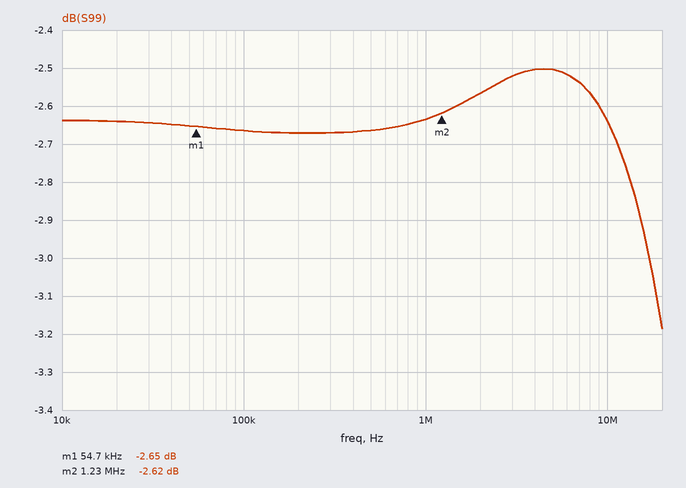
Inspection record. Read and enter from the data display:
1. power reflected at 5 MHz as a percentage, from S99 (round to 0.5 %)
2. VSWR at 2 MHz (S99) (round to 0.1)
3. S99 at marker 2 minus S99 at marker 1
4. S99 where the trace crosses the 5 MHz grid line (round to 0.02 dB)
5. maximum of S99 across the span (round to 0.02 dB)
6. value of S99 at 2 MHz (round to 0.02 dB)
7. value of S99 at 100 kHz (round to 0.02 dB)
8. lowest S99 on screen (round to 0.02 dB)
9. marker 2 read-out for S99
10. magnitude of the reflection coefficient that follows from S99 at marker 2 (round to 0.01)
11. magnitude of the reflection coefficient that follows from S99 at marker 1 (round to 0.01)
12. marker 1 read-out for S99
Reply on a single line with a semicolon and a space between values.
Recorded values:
56.0 %; 6.8; 0.03 dB; -2.50 dB; -2.50 dB; -2.56 dB; -2.66 dB; -3.18 dB; -2.62 dB; 0.74; 0.74; -2.65 dB
